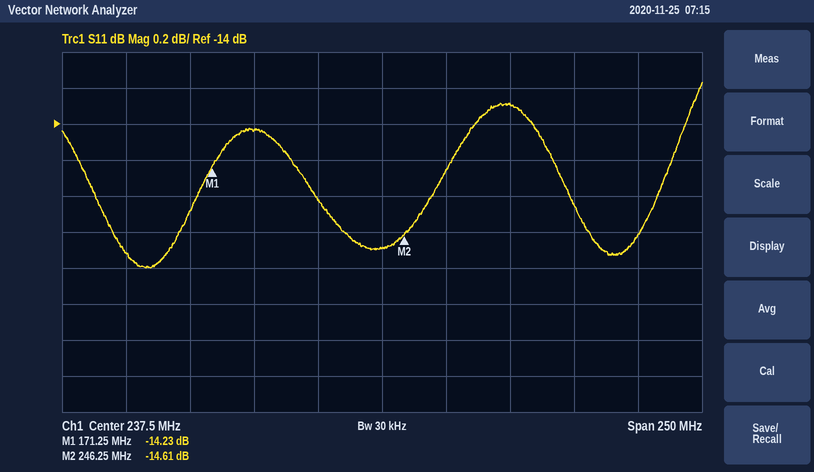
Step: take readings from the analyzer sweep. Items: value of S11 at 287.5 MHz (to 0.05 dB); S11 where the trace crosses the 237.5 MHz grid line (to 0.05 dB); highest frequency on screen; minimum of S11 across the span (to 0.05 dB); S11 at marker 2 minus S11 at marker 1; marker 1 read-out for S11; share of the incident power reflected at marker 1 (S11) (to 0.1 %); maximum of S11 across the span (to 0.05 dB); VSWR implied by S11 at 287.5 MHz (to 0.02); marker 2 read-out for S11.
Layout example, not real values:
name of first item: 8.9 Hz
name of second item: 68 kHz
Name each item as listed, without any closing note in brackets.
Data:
value of S11 at 287.5 MHz: -13.90 dB
S11 where the trace crosses the 237.5 MHz grid line: -14.70 dB
highest frequency on screen: 362.5 MHz
minimum of S11 across the span: -14.80 dB
S11 at marker 2 minus S11 at marker 1: -0.38 dB
marker 1 read-out for S11: -14.23 dB
share of the incident power reflected at marker 1 (S11): 3.8 %
maximum of S11 across the span: -13.75 dB
VSWR implied by S11 at 287.5 MHz: 1.50
marker 2 read-out for S11: -14.61 dB
